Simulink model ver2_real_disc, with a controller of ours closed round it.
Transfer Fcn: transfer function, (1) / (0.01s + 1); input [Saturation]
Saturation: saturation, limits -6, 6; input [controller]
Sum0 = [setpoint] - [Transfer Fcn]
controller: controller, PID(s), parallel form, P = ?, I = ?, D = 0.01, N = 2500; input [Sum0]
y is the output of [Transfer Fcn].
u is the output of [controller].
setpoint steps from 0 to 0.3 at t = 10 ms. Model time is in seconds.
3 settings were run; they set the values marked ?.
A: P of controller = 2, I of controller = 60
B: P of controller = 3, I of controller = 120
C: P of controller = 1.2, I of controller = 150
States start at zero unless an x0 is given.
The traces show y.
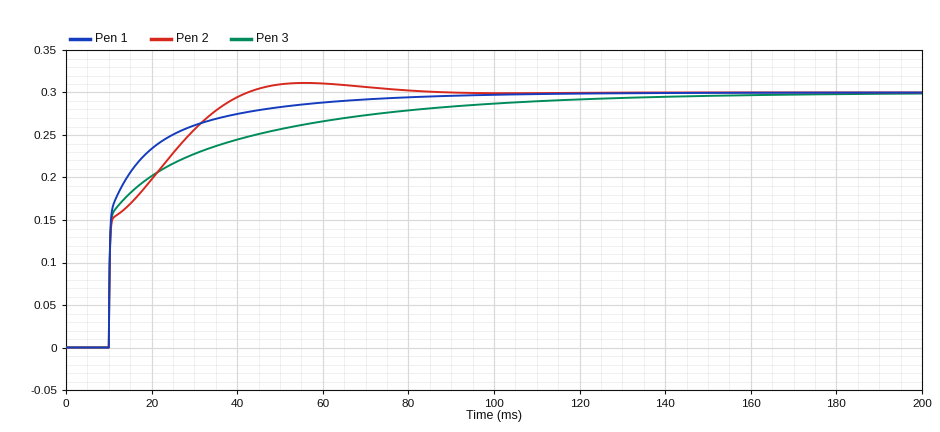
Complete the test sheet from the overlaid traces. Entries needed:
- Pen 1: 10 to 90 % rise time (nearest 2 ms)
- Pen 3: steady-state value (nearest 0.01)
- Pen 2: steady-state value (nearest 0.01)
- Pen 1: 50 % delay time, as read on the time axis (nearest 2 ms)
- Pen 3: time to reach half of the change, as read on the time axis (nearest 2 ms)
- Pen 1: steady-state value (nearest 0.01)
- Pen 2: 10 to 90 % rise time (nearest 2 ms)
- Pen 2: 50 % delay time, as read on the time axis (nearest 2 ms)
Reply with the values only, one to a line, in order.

26 ms
0.30
0.30
10 ms
10 ms
0.30
22 ms
10 ms
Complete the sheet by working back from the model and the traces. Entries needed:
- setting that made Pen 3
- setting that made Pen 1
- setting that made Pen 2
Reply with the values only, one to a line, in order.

A
B
C
